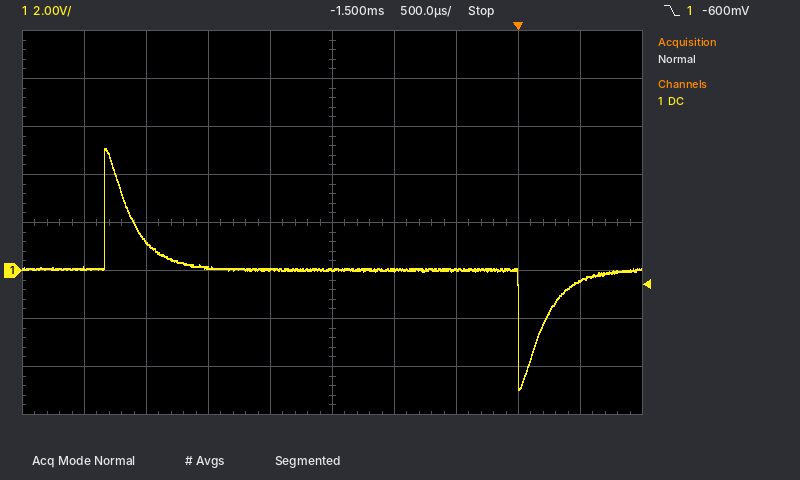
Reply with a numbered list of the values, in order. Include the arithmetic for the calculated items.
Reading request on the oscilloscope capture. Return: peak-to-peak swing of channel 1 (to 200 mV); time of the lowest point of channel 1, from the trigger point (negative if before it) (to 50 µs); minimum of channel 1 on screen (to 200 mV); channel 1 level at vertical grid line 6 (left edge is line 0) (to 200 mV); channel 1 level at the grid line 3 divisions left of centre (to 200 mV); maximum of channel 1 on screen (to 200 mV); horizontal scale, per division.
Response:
1. 5.0 V − (-5.0 V) = 10.0 V
2. 0 µs
3. -5.0 V
4. 0.0 V
5. 1.2 V
6. 5.0 V
7. 500 µs
